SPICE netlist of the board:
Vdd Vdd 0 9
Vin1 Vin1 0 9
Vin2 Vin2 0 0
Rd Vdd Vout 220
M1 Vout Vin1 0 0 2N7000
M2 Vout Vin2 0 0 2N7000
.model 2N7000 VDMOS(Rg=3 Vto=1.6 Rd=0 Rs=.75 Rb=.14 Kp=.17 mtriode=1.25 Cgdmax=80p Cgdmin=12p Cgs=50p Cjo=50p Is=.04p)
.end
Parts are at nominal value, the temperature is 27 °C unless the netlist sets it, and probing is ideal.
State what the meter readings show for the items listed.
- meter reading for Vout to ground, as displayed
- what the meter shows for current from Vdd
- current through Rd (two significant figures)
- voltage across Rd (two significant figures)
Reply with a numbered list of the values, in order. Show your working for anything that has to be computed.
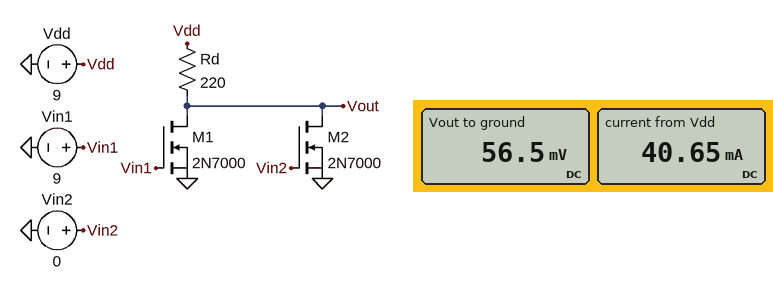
1. 56.5 mV
2. 40.65 mA
3. (9 V - 56.5 mV) / 220 Ω = 41 mA
4. 9 V - 56.5 mV = 8.9 V
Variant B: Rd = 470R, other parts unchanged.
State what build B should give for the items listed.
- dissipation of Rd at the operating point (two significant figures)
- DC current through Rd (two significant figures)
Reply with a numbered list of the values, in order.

1. 170 mW
2. 19 mA
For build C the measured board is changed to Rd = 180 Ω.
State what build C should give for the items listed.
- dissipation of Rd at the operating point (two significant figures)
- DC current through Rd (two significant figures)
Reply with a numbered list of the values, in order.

1. 440 mW
2. 50 mA
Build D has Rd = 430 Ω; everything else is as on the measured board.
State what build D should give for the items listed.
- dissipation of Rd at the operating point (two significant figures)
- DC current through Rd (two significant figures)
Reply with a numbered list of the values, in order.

1. 190 mW
2. 21 mA
